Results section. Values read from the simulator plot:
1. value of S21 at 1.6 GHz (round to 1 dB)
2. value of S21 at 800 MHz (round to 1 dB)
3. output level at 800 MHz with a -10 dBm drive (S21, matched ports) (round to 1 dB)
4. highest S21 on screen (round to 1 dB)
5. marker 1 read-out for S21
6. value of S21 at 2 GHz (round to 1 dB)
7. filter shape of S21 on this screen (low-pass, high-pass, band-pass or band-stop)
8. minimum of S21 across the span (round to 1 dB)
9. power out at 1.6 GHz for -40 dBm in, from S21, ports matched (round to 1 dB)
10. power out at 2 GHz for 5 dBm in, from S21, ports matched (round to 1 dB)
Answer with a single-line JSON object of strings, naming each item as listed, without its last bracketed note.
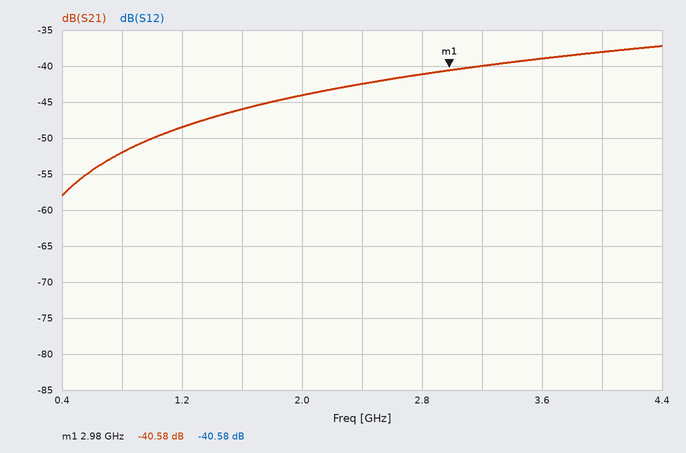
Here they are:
{"value of S21 at 1.6 GHz": "-46 dB", "value of S21 at 800 MHz": "-52 dB", "output level at 800 MHz with a -10 dBm drive (S21, matched ports)": "-62 dBm", "highest S21 on screen": "-37 dB", "marker 1 read-out for S21": "-40.58 dB", "value of S21 at 2 GHz": "-44 dB", "filter shape of S21 on this screen": "high-pass", "minimum of S21 across the span": "-58 dB", "power out at 1.6 GHz for -40 dBm in, from S21, ports matched": "-86 dBm", "power out at 2 GHz for 5 dBm in, from S21, ports matched": "-39 dBm"}
